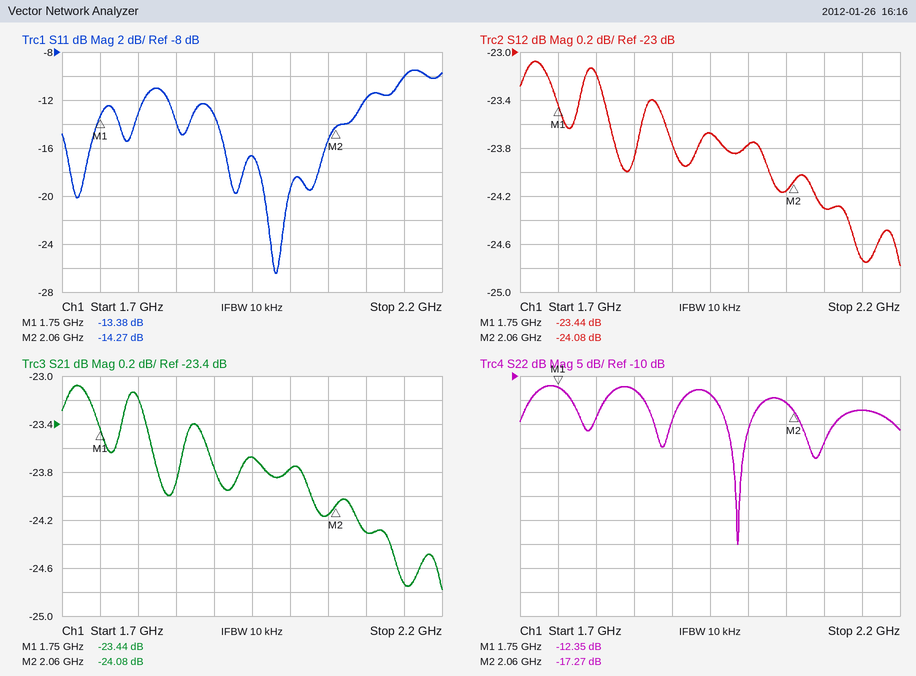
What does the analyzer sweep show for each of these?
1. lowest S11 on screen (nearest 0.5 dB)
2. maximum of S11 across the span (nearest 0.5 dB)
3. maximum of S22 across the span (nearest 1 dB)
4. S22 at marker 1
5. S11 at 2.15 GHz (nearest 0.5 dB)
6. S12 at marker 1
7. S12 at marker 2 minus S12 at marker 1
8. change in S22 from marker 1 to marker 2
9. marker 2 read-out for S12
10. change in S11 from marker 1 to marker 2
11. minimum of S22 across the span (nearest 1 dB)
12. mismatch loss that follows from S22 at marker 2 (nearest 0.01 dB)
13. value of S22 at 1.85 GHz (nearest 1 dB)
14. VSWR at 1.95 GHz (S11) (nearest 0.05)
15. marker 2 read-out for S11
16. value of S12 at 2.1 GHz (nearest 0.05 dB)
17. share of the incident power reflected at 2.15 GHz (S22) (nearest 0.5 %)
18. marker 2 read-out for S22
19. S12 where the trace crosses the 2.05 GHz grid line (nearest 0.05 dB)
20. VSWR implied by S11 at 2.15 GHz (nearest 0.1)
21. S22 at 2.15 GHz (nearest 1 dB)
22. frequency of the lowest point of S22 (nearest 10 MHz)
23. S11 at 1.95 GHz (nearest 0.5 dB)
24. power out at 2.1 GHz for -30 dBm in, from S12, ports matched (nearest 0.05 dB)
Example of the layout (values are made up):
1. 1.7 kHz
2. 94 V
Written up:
1. -26.5 dB
2. -9.5 dB
3. -12 dB
4. -12.35 dB
5. -10.0 dB
6. -23.44 dB
7. -0.64 dB
8. -4.92 dB
9. -24.08 dB
10. -0.89 dB
11. -45 dB
12. 0.08 dB
13. -13 dB
14. 1.35
15. -14.27 dB
16. -24.30 dB
17. 2.0 %
18. -17.27 dB
19. -24.15 dB
20. 1.9
21. -17 dB
22. 1.99 GHz
23. -16.5 dB
24. -54.30 dBm
